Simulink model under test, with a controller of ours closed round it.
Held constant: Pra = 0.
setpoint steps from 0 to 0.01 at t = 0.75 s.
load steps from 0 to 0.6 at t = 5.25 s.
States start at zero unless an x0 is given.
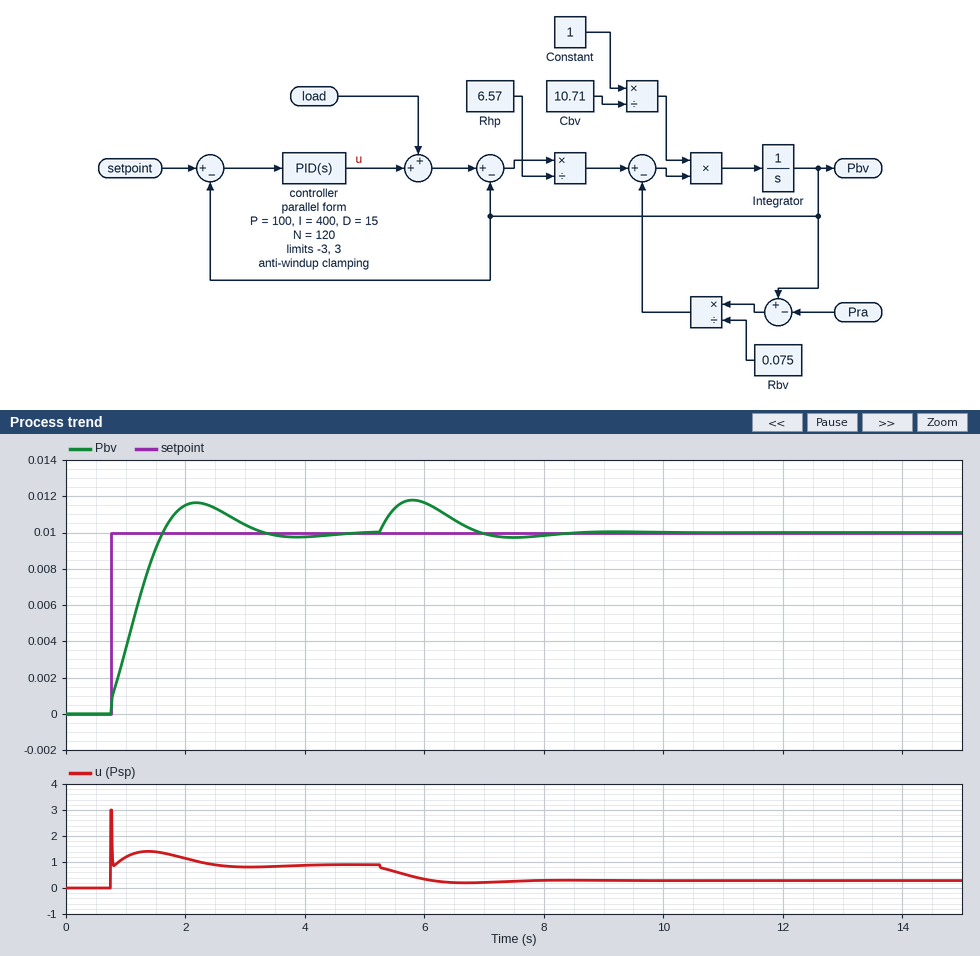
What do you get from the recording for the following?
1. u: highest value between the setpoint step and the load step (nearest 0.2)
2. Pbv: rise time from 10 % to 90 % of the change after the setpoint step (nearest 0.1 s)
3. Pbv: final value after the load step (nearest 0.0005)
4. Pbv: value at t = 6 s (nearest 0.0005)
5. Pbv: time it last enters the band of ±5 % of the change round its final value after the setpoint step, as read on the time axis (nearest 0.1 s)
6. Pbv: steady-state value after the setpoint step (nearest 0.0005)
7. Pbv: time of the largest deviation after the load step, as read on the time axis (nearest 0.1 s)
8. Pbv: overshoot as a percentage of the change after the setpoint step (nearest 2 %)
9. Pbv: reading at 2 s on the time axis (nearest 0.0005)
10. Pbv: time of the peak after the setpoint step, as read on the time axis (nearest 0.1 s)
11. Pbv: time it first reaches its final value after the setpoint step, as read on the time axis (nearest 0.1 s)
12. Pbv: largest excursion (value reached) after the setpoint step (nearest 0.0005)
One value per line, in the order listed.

3.0
0.7 s
0.0100
0.0115
3.0 s
0.0100
5.8 s
16 %
0.0115
2.2 s
1.6 s
0.0115
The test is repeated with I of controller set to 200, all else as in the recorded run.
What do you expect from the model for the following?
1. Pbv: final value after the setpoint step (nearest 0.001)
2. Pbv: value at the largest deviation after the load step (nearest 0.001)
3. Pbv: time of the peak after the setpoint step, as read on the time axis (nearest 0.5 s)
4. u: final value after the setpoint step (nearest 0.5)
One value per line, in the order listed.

0.010
0.012
3.0 s
1.0
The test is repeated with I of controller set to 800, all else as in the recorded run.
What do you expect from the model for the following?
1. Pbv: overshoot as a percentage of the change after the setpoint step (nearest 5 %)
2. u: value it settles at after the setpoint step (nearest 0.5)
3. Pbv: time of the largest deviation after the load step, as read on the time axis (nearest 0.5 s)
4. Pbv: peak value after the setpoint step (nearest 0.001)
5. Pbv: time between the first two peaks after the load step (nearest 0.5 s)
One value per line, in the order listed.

30 %
1.0
5.5 s
0.013
2.0 s
